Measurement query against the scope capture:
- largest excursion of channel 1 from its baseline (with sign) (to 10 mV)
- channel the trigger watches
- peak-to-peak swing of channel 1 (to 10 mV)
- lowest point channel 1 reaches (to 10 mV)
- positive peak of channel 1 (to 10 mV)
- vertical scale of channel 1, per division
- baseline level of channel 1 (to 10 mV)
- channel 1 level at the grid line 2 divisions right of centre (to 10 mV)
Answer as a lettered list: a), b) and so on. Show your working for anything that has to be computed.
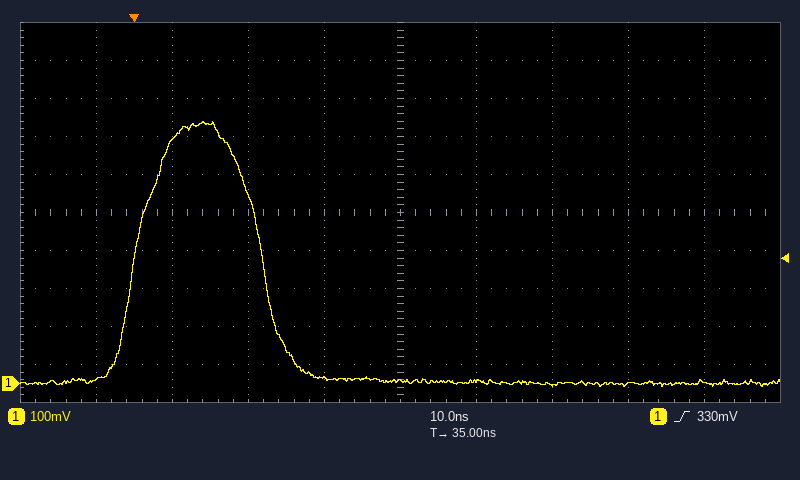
a) 690 mV − (0 mV) = +690 mV
b) channel 1
c) 690 mV − (-10 mV) = 700 mV
d) -10 mV
e) 690 mV
f) 100 mV
g) 0 mV
h) 0 mV
